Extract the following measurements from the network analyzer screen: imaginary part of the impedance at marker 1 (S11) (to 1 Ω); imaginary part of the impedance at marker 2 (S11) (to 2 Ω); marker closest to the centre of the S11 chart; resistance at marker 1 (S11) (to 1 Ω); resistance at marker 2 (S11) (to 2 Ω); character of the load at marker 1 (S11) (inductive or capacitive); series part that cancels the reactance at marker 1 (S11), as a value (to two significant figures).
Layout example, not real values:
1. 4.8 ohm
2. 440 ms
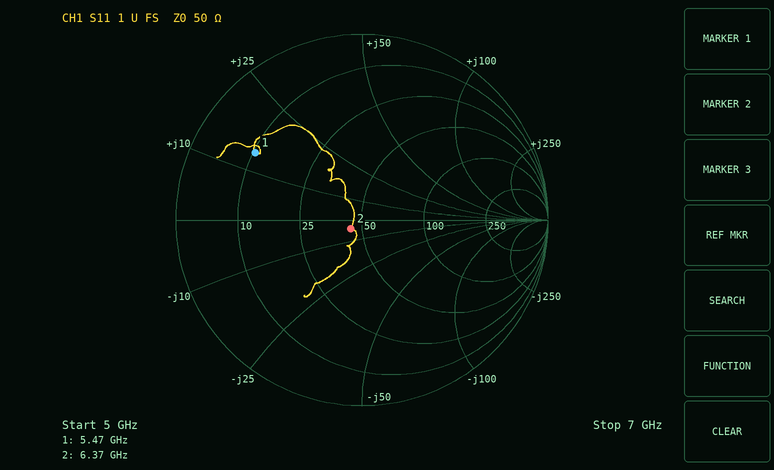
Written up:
1. +14 Ω
2. -4 Ω
3. marker 2
4. 10 Ω
5. 44 Ω
6. inductive
7. 2.1 pF
